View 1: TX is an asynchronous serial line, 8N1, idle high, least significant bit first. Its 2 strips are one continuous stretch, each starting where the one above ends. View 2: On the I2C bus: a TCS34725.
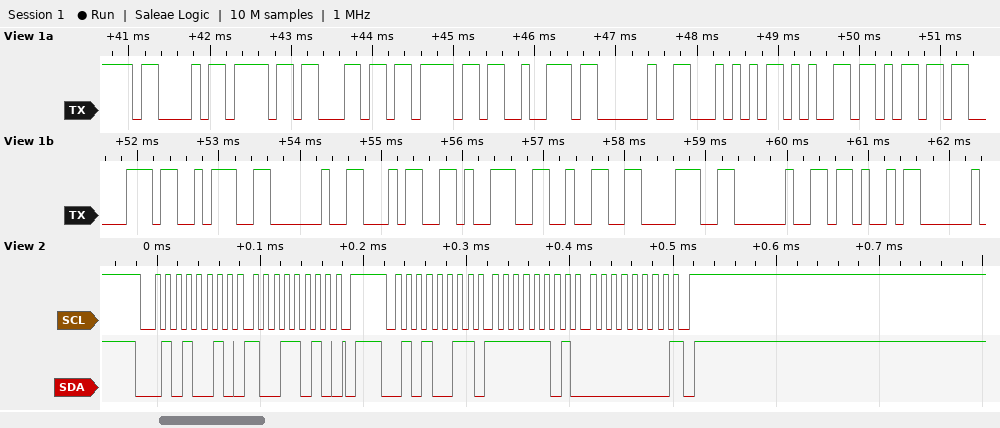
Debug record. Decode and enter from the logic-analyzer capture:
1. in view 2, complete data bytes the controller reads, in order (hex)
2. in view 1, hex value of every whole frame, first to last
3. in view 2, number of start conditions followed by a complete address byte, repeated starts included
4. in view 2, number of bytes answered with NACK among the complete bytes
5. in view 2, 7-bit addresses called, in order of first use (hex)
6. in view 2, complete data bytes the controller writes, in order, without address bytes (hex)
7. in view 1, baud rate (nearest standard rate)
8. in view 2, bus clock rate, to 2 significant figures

FD 00
43 6F 6C 6F 72 20 54 65 6D 70 3A 20 34 39 32 38 20 4B
2
1
0x29
9A
9600 baud
100 kHz
